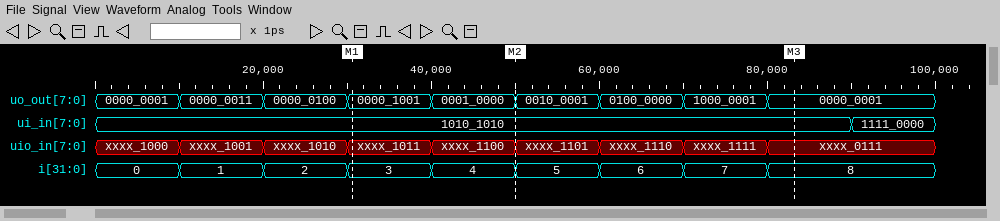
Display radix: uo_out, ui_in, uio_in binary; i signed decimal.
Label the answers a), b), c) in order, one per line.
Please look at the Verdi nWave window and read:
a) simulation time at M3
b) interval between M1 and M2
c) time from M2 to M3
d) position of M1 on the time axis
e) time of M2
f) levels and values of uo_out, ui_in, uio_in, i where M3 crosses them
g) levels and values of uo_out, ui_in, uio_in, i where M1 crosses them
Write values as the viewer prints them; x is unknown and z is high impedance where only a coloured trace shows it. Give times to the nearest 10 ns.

a) 80 ns
b) 20 ns
c) 30 ns
d) 30 ns
e) 50 ns
f) uo_out=0000_0001, ui_in=1010_1010, uio_in=xxxx_0111, i=8
g) uo_out=0000_1001, ui_in=1010_1010, uio_in=xxxx_1011, i=3
